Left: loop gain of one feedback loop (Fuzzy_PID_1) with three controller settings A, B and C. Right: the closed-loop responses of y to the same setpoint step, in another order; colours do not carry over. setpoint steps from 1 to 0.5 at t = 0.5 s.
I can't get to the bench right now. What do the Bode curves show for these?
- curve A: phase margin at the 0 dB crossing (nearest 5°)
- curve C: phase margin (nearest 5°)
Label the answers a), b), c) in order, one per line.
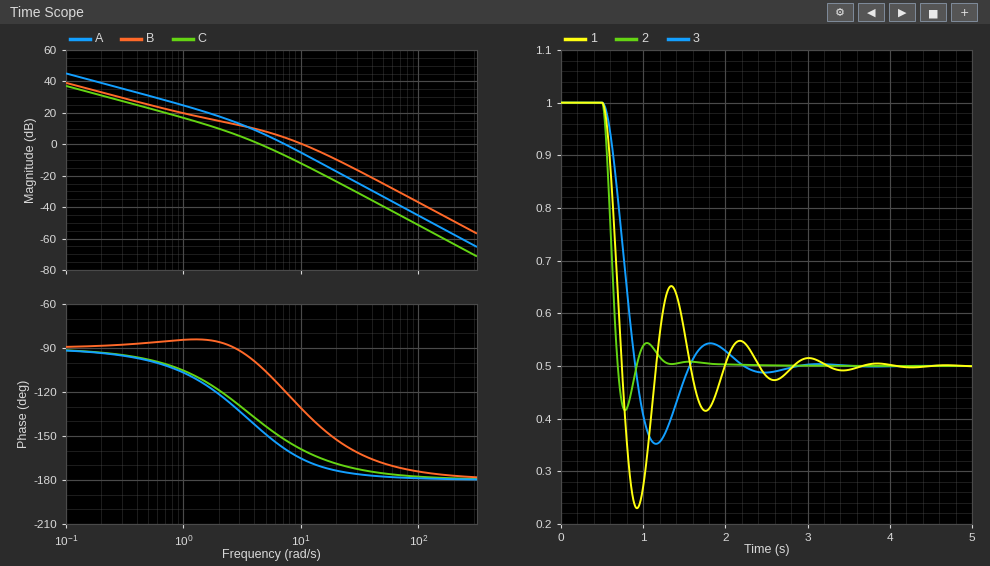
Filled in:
a) 20°
b) 40°
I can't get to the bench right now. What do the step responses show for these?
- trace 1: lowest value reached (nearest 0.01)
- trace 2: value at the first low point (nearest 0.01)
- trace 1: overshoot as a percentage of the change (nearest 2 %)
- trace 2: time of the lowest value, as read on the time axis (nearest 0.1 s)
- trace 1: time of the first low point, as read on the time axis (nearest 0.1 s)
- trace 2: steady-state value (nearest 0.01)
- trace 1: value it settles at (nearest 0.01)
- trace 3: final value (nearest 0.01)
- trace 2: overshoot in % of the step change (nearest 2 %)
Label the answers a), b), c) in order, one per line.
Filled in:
a) 0.23
b) 0.42
c) 54 %
d) 0.8 s
e) 0.9 s
f) 0.50
g) 0.50
h) 0.50
i) 16 %
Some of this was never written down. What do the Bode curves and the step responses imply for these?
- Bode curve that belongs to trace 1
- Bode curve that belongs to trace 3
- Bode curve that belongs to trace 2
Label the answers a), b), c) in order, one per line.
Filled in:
a) A
b) C
c) B
